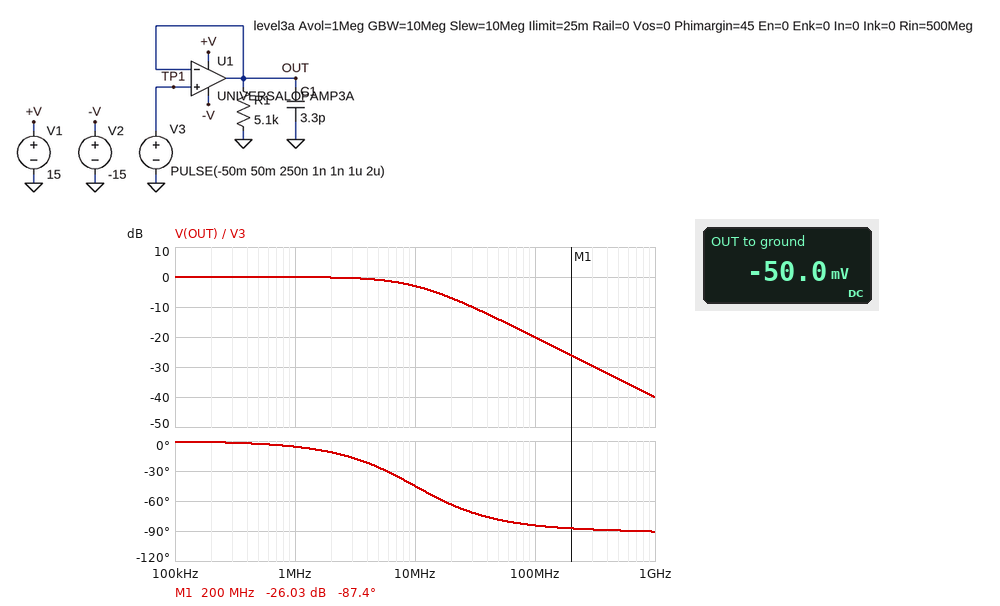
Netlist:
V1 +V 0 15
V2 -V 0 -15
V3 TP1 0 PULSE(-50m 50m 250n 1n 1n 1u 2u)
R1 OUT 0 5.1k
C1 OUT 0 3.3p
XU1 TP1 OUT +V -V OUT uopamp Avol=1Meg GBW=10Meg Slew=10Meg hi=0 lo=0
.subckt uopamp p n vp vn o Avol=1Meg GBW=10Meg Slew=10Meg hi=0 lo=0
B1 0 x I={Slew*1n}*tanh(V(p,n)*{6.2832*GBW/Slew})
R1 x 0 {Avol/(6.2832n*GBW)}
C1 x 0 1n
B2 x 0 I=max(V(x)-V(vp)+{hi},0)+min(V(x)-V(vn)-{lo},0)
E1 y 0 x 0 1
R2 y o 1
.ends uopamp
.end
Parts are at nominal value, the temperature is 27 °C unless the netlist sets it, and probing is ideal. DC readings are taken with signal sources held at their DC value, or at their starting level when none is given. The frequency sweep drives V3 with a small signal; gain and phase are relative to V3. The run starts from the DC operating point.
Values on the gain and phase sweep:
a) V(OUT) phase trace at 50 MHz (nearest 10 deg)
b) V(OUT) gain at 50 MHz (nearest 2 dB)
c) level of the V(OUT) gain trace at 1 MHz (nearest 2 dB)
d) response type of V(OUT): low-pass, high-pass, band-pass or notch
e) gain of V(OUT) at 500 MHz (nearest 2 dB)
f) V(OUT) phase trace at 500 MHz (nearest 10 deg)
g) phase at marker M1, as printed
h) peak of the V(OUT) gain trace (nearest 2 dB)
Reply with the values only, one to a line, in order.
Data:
-80 deg
-14 dB
0 dB
low-pass
-34 dB
-90 deg
-87.4 deg
0 dB
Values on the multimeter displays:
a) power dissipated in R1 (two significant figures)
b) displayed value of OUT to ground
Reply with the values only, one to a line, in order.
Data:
490 nW
-50.0 mV
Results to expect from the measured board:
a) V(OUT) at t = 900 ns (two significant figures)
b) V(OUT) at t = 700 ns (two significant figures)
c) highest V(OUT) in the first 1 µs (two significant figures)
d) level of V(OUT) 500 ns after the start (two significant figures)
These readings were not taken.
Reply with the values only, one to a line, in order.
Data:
50 mV
50 mV
50 mV
50 mV
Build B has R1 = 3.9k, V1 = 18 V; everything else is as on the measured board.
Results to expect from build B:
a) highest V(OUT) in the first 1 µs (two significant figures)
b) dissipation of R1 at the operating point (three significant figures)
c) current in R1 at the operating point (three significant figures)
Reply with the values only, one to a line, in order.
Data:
50 mV
641 nW
12.8 µA
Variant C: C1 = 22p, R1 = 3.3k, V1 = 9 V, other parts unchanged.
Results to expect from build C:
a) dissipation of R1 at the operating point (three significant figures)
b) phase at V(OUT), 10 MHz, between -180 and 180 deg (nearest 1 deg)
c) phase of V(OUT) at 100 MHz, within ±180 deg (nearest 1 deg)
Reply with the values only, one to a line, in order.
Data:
758 nW
-45 deg
-85 deg
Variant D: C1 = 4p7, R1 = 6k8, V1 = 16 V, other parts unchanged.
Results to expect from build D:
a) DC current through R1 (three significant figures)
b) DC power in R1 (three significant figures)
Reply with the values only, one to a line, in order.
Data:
7.35 µA
368 nW
